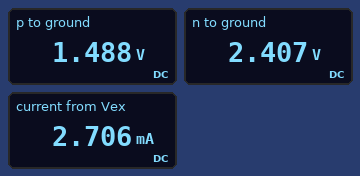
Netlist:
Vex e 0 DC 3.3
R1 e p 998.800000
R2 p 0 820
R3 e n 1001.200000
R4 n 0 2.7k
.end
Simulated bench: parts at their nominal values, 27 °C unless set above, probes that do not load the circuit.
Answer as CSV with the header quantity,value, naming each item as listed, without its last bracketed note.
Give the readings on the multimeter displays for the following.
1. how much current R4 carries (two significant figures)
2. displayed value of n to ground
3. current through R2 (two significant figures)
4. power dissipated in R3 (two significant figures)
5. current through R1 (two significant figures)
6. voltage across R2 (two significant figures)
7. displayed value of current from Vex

quantity,value
how much current R4 carries,890 µA
displayed value of n to ground,2.407 V
current through R2,1.8 mA
power dissipated in R3,800 µW
current through R1,1.8 mA
voltage across R2,1.5 V
displayed value of current from Vex,2.706 mA
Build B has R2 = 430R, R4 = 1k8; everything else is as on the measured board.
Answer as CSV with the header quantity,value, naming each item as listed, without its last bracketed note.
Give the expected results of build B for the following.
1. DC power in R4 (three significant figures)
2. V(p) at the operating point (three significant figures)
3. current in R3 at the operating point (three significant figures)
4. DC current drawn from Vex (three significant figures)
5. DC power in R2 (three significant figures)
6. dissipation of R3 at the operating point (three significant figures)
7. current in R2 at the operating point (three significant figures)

quantity,value
DC power in R4,2.50 mW
V(p) at the operating point,993 mV
current in R3 at the operating point,1.18 mA
DC current drawn from Vex,3.49 mA
DC power in R2,2.29 mW
dissipation of R3 at the operating point,1.39 mW
current in R2 at the operating point,2.31 mA
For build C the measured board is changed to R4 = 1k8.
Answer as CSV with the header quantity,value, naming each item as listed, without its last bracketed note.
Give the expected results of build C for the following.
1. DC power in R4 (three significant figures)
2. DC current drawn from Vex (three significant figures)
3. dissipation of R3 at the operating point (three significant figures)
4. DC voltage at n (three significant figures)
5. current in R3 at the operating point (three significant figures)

quantity,value
DC power in R4,2.50 mW
DC current drawn from Vex,2.99 mA
dissipation of R3 at the operating point,1.39 mW
DC voltage at n,2.12 V
current in R3 at the operating point,1.18 mA
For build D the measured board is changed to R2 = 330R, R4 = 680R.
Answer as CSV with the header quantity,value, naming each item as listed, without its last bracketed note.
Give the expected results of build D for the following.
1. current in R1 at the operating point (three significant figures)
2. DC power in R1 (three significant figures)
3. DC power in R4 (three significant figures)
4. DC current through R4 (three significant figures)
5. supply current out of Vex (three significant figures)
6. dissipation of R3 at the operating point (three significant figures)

quantity,value
current in R1 at the operating point,2.48 mA
DC power in R1,6.16 mW
DC power in R4,2.62 mW
DC current through R4,1.96 mA
supply current out of Vex,4.45 mA
dissipation of R3 at the operating point,3.86 mW
